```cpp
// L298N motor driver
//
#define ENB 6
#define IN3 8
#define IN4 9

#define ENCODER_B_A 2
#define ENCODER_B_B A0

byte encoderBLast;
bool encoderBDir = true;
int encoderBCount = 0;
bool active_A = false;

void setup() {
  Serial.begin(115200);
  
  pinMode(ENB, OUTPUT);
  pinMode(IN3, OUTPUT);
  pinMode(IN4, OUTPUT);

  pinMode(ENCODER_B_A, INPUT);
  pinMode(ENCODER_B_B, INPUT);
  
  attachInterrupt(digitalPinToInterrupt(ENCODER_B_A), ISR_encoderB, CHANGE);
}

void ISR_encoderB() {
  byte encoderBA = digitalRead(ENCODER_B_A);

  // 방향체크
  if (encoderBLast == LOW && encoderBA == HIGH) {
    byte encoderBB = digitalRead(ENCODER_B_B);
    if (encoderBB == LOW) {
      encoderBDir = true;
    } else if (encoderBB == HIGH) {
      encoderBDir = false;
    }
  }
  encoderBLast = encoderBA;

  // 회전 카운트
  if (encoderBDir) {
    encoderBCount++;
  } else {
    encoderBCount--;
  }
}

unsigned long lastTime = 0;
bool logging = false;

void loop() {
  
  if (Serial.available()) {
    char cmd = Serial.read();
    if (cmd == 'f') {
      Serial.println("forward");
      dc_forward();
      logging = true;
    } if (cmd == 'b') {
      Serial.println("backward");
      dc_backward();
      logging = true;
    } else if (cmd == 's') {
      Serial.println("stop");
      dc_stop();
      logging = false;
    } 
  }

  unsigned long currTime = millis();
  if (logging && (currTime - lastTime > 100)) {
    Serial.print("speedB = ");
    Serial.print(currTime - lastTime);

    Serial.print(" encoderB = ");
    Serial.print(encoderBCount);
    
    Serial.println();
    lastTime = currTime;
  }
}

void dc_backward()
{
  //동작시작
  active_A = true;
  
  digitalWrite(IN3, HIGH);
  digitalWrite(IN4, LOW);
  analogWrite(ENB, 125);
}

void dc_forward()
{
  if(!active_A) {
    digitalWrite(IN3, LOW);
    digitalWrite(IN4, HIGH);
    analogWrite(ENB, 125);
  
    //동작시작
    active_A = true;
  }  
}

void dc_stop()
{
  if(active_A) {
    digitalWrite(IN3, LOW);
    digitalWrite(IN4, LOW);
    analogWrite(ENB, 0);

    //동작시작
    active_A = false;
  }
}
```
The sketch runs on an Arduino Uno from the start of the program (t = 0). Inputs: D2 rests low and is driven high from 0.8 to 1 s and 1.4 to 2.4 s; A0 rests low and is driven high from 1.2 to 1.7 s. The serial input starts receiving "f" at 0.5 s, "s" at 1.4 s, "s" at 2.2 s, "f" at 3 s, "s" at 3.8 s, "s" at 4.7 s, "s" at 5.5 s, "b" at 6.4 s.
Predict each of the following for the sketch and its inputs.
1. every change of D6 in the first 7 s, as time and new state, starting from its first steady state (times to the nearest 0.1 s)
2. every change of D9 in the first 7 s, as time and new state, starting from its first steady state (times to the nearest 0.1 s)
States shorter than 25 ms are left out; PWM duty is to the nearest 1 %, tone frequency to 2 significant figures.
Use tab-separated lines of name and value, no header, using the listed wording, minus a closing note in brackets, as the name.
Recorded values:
every change of D6 in the first 7 s, as time and new state, starting from its first steady state	0 s low; 0.5 s PWM 49 %; 1.4 s low; 3 s PWM 49 %; 3.8 s low; 6.4 s PWM 49 %
every change of D9 in the first 7 s, as time and new state, starting from its first steady state	0 s low; 0.5 s high; 1.4 s low; 3 s high; 3.8 s low
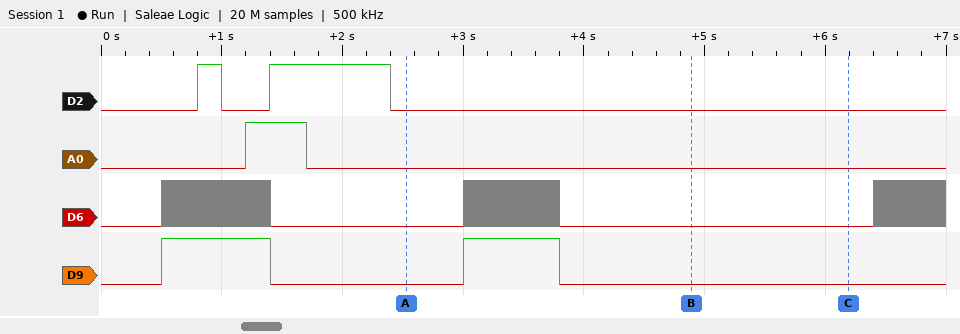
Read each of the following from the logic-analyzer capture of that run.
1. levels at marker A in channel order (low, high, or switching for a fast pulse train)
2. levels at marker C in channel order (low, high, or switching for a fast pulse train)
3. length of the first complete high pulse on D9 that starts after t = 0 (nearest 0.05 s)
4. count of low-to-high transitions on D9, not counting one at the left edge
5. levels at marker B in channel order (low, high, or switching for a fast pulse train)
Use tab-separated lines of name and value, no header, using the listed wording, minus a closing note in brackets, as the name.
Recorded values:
levels at marker A in channel order	D2 low, A0 low, D6 low, D9 low
levels at marker C in channel order	D2 low, A0 low, D6 low, D9 low
length of the first complete high pulse on D9 that starts after t = 0	0.90 s
count of low-to-high transitions on D9, not counting one at the left edge	2
levels at marker B in channel order	D2 low, A0 low, D6 low, D9 low
